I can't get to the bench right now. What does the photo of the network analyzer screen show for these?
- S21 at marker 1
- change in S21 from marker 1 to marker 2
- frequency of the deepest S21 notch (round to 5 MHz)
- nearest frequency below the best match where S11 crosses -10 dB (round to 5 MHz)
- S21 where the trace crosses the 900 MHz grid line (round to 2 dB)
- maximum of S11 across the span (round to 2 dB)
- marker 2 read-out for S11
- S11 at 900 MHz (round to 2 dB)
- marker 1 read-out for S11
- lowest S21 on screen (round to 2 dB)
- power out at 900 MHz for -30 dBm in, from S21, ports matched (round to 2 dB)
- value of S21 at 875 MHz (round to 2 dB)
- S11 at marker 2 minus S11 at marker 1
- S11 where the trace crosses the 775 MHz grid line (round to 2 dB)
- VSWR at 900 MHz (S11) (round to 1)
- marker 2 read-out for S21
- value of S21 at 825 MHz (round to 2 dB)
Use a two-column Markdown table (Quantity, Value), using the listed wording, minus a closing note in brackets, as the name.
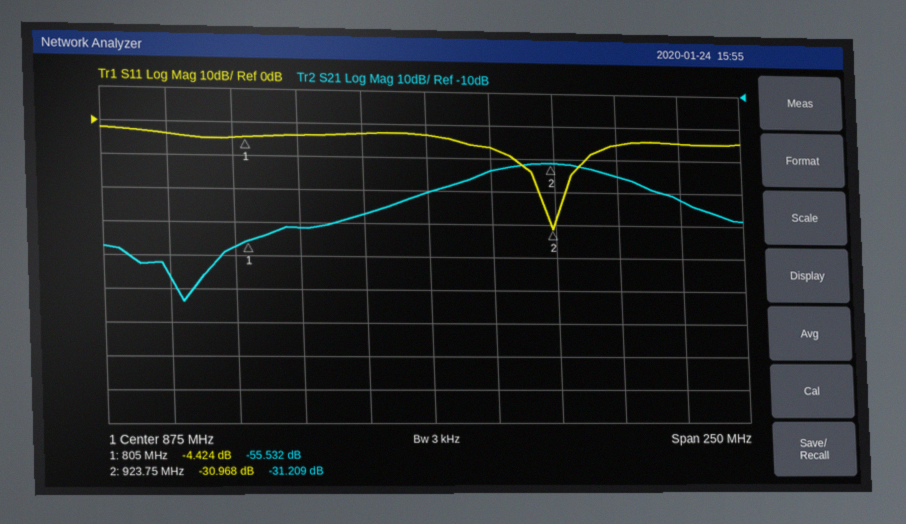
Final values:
| Quantity | Value |
|---|---|
| S21 at marker 1 | -55.532 dB |
| change in S21 from marker 1 to marker 2 | 24.323 dB |
| frequency of the deepest S21 notch | 780 MHz |
| nearest frequency below the best match where S11 crosses -10 dB | 910 MHz |
| S21 where the trace crosses the 900 MHz grid line | -34 dB |
| maximum of S11 across the span | -2 dB |
| marker 2 read-out for S11 | -30.968 dB |
| S11 at 900 MHz | -6 dB |
| marker 1 read-out for S11 | -4.424 dB |
| lowest S21 on screen | -74 dB |
| power out at 900 MHz for -30 dBm in, from S21, ports matched | -64 dBm |
| value of S21 at 875 MHz | -40 dB |
| S11 at marker 2 minus S11 at marker 1 | -26.544 dB |
| S11 where the trace crosses the 775 MHz grid line | -4 dB |
| VSWR at 900 MHz (S11) | 3 |
| marker 2 read-out for S21 | -31.209 dB |
| value of S21 at 825 MHz | -52 dB |
